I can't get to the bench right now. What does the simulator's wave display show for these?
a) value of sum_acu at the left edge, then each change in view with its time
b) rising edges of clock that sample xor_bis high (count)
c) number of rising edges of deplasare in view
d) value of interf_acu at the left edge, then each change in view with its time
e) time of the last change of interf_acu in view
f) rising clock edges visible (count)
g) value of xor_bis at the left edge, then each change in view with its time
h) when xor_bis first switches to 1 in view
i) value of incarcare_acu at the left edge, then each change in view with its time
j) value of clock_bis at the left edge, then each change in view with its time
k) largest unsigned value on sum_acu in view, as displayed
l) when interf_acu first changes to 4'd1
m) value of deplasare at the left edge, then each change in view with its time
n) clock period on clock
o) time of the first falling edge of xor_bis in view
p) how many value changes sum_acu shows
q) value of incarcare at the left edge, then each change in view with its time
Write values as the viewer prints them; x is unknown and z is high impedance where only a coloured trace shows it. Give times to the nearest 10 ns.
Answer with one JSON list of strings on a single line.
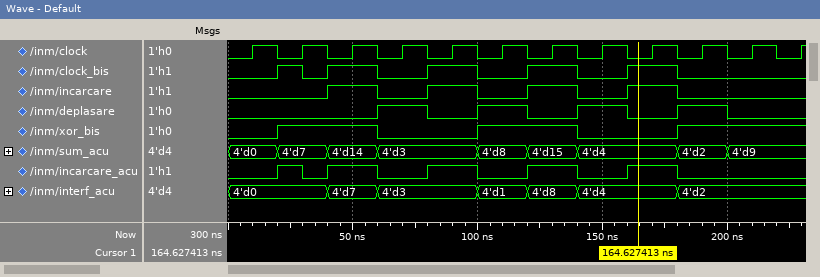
["4'd0, 4'd7 at 20 ns, 4'd14 at 40 ns, 4'd3 at 60 ns, 4'd8 at 100 ns, 4'd15 at 120 ns, 4'd4 at 140 ns, 4'd2 at 180 ns, 4'd9 at 200 ns", "7", "4", "4'd0, 4'd7 at 40 ns, 4'd3 at 60 ns, 4'd1 at 100 ns, 4'd8 at 120 ns, 4'd4 at 140 ns, 4'd2 at 180 ns", "180 ns", "12", "0, 1 at 20 ns, 0 at 60 ns, 1 at 100 ns, 0 at 140 ns, 1 at 180 ns", "20 ns", "0, 1 at 20 ns, 0 at 30 ns, 1 at 40 ns, 0 at 60 ns, 1 at 80 ns, 0 at 100 ns, 1 at 120 ns, 0 at 140 ns, 1 at 160 ns, 0 at 180 ns", "0, 1 at 20 ns, 0 at 30 ns, 1 at 40 ns, 0 at 60 ns, 1 at 80 ns, 0 at 100 ns, 1 at 120 ns, 0 at 140 ns, 1 at 160 ns, 0 at 180 ns", "4'd15", "100 ns", "0, 1 at 60 ns, 0 at 80 ns, 1 at 100 ns, 0 at 120 ns, 1 at 140 ns, 0 at 160 ns, 1 at 180 ns, 0 at 200 ns", "20 ns", "60 ns", "8", "0, 1 at 40 ns, 0 at 60 ns, 1 at 80 ns, 0 at 100 ns, 1 at 120 ns, 0 at 140 ns, 1 at 160 ns, 0 at 180 ns"]
